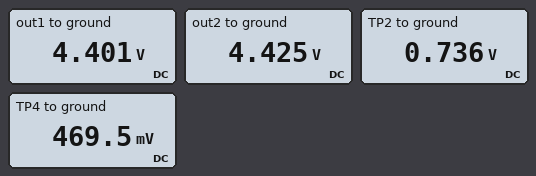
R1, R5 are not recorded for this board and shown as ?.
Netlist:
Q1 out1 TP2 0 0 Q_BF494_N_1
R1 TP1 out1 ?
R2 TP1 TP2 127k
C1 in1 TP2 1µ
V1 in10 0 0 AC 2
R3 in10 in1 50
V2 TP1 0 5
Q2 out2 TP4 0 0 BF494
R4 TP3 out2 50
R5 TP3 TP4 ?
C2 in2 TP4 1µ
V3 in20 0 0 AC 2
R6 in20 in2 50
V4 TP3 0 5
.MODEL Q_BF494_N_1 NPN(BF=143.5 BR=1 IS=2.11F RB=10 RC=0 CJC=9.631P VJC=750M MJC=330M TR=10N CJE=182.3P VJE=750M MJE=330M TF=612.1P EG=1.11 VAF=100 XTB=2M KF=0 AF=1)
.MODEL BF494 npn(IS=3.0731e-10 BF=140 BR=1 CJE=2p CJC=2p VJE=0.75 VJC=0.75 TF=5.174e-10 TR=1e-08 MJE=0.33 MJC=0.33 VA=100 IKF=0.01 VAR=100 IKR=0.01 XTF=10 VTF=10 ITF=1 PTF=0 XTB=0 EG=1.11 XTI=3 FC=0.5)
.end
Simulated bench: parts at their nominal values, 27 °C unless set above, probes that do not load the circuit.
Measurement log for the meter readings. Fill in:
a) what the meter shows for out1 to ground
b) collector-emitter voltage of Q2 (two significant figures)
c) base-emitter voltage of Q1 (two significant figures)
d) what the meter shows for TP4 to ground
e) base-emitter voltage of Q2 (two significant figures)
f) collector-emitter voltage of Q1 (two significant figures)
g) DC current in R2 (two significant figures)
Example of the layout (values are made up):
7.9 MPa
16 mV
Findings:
4.401 V
4.4 V
740 mV
469.5 mV
470 mV
4.4 V
34 µA
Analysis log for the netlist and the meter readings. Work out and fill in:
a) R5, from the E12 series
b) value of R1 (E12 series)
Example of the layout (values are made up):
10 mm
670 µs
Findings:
27 kΩ
120 Ω
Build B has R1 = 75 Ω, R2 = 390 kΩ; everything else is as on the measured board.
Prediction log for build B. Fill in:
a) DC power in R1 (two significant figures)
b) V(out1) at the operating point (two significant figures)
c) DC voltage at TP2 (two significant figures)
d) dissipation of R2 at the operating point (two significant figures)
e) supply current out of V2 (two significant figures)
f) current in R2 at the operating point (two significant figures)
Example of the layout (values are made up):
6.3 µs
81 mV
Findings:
200 µW
4.9 V
710 mV
47 µW
1.7 mA
11 µA
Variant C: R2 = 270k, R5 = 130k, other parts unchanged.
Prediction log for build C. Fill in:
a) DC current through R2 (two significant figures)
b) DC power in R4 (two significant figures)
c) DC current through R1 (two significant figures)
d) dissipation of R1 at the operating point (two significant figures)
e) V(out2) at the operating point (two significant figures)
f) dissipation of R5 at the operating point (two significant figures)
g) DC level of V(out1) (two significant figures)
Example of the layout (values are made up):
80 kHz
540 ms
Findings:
16 µA
710 µW
2.4 mA
670 µW
4.8 V
160 µW
4.7 V
